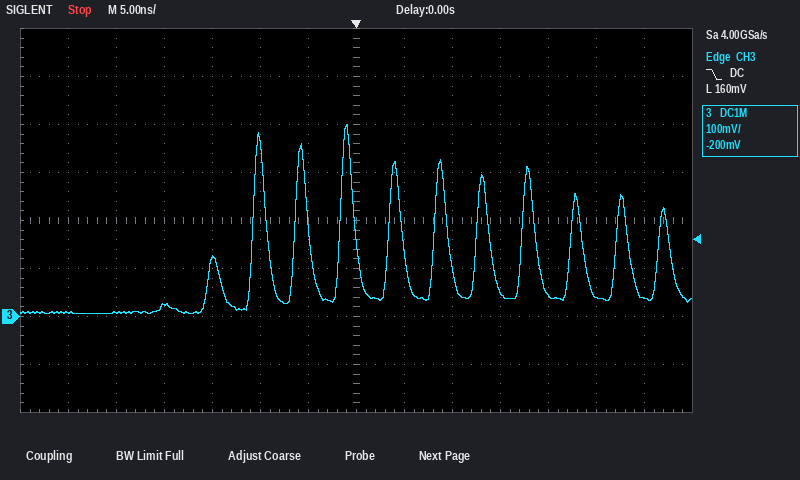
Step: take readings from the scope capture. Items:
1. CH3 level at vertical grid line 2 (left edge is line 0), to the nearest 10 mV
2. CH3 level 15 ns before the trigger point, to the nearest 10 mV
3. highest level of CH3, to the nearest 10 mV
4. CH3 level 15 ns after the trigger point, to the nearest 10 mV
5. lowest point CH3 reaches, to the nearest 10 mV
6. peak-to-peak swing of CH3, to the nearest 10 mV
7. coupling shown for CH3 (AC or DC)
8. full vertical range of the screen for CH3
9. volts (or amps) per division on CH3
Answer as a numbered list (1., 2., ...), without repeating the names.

1. 10 mV
2. 120 mV
3. 400 mV
4. 50 mV
5. 10 mV
6. 390 mV
7. DC
8. 800 mV
9. 100 mV
